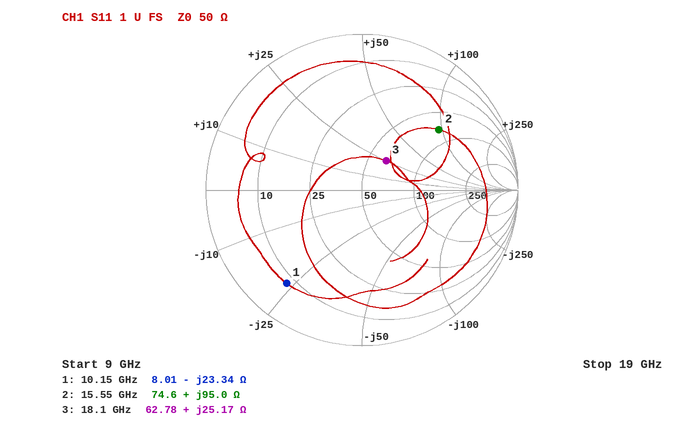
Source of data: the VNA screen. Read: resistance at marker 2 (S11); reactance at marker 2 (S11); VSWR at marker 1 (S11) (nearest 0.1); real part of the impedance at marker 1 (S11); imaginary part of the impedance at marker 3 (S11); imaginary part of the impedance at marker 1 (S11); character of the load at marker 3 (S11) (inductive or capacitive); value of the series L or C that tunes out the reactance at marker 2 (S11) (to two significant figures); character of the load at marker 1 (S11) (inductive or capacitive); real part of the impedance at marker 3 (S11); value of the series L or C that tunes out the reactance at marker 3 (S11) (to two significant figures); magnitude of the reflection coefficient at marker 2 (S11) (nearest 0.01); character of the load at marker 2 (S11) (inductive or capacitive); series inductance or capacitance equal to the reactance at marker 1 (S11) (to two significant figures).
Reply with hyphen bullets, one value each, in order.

- 74.6 Ω
- +95.0 Ω
- 7.6
- 8.01 Ω
- +25.17 Ω
- -23.34 Ω
- inductive
- 110 fF
- capacitive
- 62.78 Ω
- 350 fF
- 0.63
- inductive
- 670 fF
